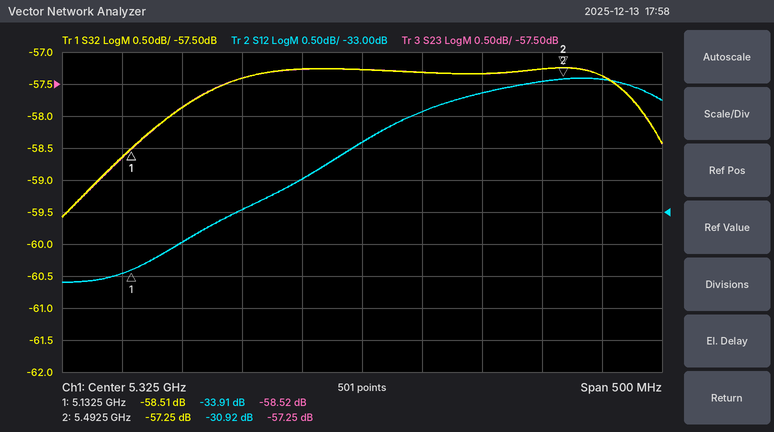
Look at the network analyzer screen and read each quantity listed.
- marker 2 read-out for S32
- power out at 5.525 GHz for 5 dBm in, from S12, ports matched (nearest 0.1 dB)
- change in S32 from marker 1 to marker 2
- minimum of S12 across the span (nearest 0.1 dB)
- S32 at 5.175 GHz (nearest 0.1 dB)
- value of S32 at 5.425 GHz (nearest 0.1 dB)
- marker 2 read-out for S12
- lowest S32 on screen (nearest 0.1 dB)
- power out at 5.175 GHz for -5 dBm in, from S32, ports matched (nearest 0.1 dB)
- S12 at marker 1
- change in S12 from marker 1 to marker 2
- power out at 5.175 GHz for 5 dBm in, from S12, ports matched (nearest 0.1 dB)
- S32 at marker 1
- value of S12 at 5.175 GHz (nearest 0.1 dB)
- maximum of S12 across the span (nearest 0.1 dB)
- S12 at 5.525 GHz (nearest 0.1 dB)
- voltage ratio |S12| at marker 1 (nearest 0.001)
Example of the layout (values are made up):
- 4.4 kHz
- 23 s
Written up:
- -57.25 dB
- -25.9 dBm
- 1.26 dB
- -34.1 dB
- -57.9 dB
- -57.3 dB
- -30.92 dB
- -59.6 dB
- -62.9 dBm
- -33.91 dB
- 2.99 dB
- -28.5 dBm
- -58.51 dB
- -33.5 dB
- -30.9 dB
- -30.9 dB
- 0.020
